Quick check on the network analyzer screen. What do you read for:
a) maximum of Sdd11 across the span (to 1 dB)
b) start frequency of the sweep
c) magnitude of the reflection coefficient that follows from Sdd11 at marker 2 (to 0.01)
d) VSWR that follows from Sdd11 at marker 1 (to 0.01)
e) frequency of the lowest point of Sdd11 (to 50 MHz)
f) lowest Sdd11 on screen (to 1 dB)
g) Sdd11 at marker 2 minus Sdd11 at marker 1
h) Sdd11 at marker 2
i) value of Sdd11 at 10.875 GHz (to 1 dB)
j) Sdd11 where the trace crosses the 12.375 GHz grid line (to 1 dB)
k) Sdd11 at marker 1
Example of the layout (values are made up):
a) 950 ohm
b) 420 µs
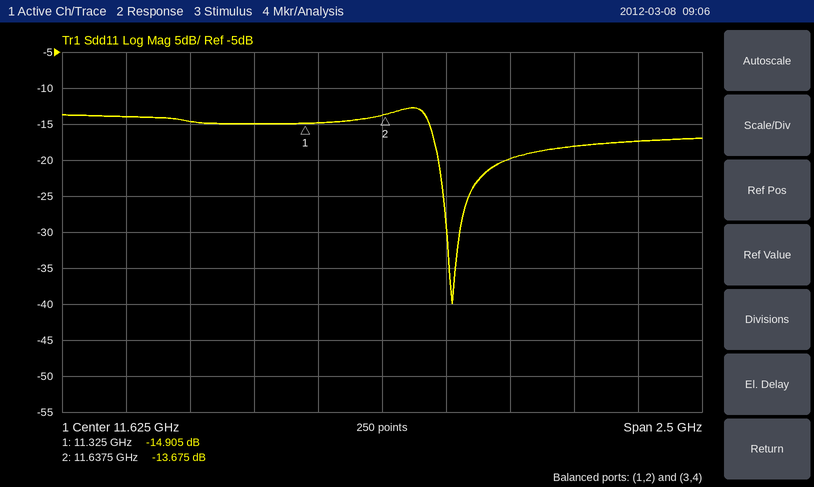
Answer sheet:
a) -13 dB
b) 10.375 GHz
c) 0.21
d) 1.44
e) 11.90 GHz
f) -40 dB
g) 1.230 dB
h) -13.675 dB
i) -15 dB
j) -18 dB
k) -14.905 dB
